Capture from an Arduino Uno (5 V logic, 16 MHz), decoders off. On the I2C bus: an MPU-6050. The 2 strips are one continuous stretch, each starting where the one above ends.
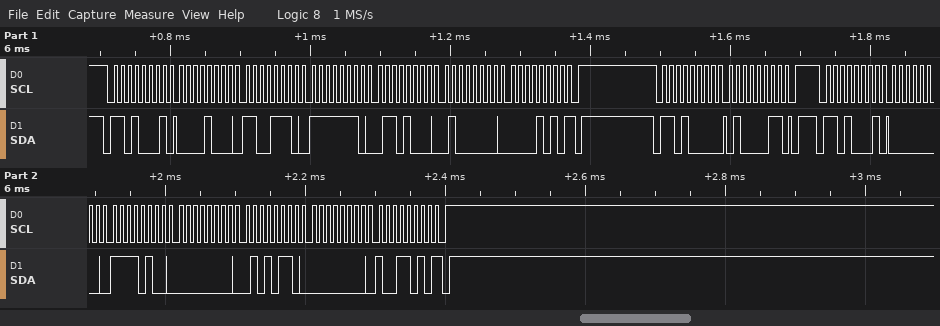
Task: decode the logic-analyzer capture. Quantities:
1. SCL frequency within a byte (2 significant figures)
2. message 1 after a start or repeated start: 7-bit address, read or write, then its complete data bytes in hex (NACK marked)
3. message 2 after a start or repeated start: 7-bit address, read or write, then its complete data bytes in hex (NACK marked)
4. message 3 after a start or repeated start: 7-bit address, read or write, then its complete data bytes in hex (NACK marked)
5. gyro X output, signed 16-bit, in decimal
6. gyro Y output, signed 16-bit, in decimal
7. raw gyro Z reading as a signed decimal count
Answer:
100 kHz
0x68 read: 08 CE FE 68 40 0A NACK
0x68 write: 43
0x68 read: 00 F4 00 56 00 9A NACK
244
86
154
